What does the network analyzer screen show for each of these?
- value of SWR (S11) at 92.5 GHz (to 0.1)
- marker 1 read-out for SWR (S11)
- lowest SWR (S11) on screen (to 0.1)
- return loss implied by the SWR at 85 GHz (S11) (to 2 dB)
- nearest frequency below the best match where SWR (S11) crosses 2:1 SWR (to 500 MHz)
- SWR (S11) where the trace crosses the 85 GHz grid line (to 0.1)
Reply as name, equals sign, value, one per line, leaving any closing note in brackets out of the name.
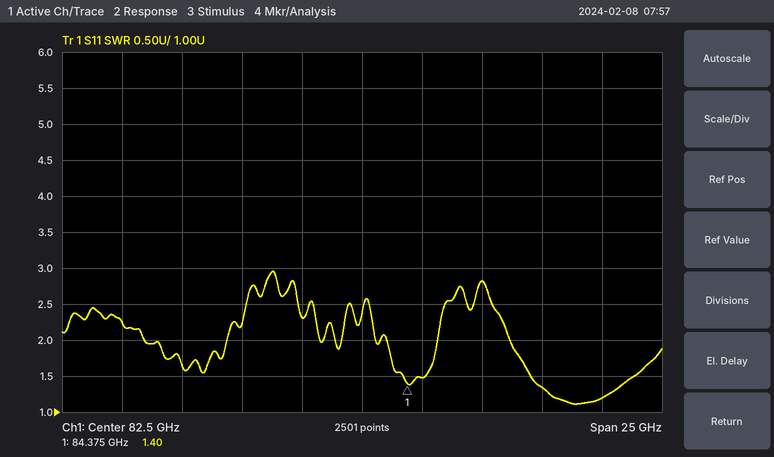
value of SWR (S11) at 92.5 GHz = 1.2
marker 1 read-out for SWR = 1.40
lowest SWR (S11) on screen = 1.1
return loss implied by the SWR at 85 GHz (S11) = 14 dB
nearest frequency below the best match where SWR (S11) crosses 2:1 SWR = 88.5 GHz
SWR (S11) where the trace crosses the 85 GHz grid line = 1.5
